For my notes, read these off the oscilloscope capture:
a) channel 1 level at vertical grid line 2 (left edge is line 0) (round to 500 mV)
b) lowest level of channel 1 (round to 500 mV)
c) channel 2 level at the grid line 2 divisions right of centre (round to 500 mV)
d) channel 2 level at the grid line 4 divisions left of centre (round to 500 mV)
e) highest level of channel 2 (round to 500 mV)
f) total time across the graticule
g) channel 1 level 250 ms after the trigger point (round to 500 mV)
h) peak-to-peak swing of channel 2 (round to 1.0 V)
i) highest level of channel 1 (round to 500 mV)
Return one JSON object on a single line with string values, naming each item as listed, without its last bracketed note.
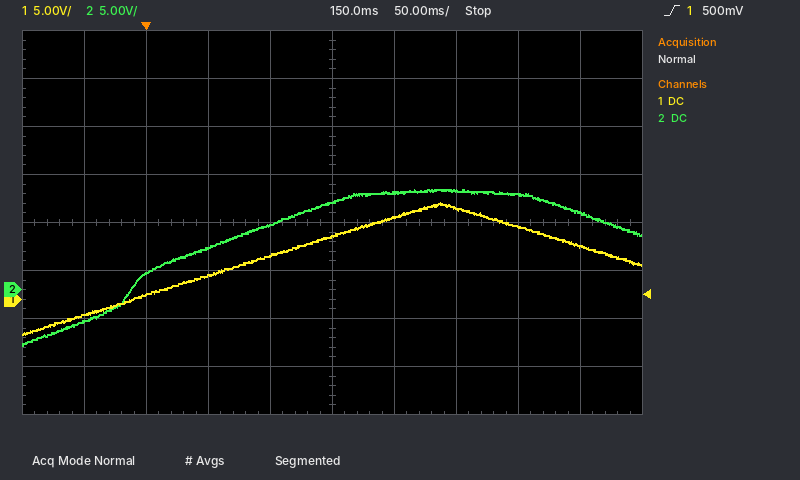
{"channel 1 level at vertical grid line 2 (left edge is line 0)": "500 mV", "lowest level of channel 1": "-3.5 V", "channel 2 level at the grid line 2 divisions right of centre": "10.5 V", "channel 2 level at the grid line 4 divisions left of centre": "-3.5 V", "highest level of channel 2": "10.5 V", "total time across the graticule": "500 ms", "channel 1 level 250 ms after the trigger point": "9.5 V", "peak-to-peak swing of channel 2": "16.0 V", "highest level of channel 1": "10.0 V"}
